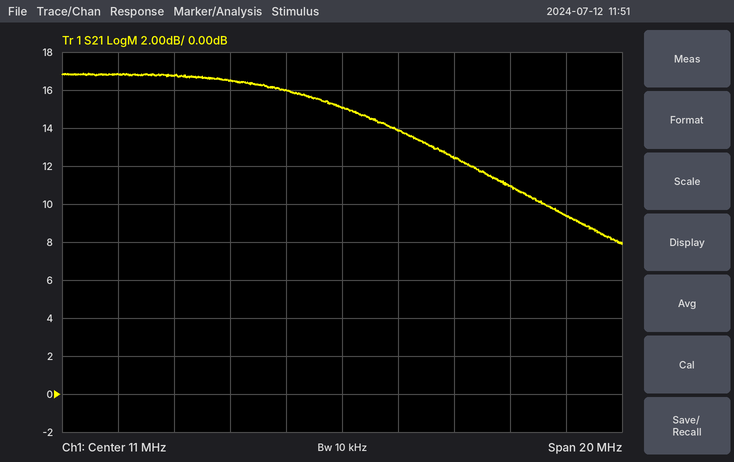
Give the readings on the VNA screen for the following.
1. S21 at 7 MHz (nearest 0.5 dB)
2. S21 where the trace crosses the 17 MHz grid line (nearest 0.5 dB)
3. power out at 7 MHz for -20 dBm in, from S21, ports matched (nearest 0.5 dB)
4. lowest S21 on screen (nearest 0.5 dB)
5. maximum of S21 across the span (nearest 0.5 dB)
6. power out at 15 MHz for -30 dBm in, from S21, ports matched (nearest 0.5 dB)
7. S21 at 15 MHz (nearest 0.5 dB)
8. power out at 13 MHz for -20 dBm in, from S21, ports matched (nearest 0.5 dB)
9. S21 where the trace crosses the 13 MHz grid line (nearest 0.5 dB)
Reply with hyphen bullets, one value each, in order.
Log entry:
- 16.5 dB
- 11.0 dB
- -3.5 dBm
- 8.0 dB
- 17.0 dB
- -17.5 dBm
- 12.5 dB
- -6.0 dBm
- 14.0 dB
